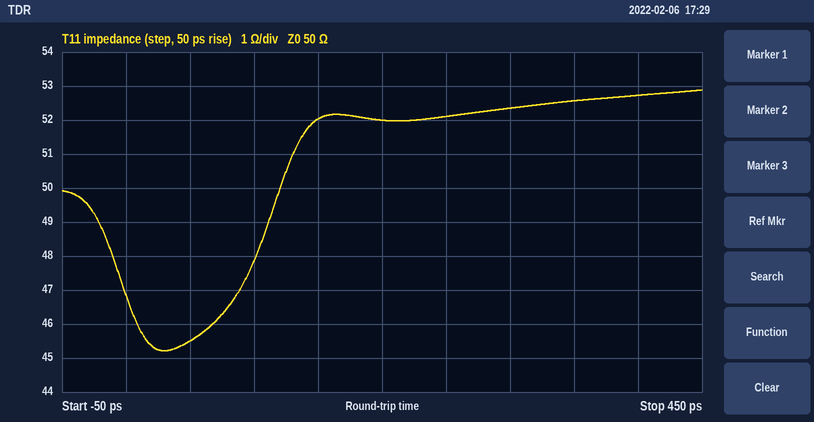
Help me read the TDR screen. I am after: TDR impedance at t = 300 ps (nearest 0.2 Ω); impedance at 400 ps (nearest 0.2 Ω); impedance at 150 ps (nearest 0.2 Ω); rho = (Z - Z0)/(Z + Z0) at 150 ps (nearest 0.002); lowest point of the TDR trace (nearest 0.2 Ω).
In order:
52.4 Ω
52.8 Ω
52.0 Ω
+0.020
45.2 Ω
